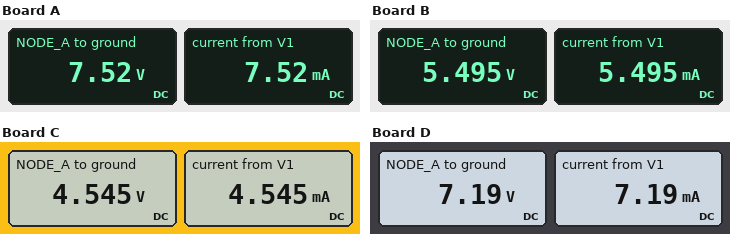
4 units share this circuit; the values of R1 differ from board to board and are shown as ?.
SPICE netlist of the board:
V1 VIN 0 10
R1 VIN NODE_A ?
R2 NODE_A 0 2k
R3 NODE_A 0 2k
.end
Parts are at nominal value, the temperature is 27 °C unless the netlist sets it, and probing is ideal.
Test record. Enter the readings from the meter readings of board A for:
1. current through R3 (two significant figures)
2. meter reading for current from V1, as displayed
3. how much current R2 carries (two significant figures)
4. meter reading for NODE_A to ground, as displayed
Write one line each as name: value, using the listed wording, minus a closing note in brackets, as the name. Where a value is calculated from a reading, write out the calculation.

current through R3: (7.52 V) / 2 kΩ = 3.8 mA
meter reading for current from V1, as displayed: 7.52 mA
how much current R2 carries: (7.52 V) / 2 kΩ = 3.8 mA
meter reading for NODE_A to ground, as displayed: 7.52 V
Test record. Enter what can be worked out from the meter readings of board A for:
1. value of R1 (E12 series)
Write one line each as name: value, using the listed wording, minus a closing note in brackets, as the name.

value of R1: 330 Ω
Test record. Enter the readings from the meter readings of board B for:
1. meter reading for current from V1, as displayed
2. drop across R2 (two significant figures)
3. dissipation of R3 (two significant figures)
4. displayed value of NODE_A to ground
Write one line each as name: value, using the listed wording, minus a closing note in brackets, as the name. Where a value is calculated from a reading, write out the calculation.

meter reading for current from V1, as displayed: 5.495 mA
drop across R2: 5.495 V = 5.5 V
dissipation of R3: (5.495 V)^2 / 2 kΩ = 15 mW
displayed value of NODE_A to ground: 5.495 V
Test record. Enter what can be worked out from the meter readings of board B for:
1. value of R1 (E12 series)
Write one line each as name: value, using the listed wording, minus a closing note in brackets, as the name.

value of R1: 820 Ω
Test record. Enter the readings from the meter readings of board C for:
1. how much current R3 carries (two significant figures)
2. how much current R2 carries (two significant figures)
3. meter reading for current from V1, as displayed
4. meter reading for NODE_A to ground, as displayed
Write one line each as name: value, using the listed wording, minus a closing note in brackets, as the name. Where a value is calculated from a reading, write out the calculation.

how much current R3 carries: (4.545 V) / 2 kΩ = 2.3 mA
how much current R2 carries: (4.545 V) / 2 kΩ = 2.3 mA
meter reading for current from V1, as displayed: 4.545 mA
meter reading for NODE_A to ground, as displayed: 4.545 V
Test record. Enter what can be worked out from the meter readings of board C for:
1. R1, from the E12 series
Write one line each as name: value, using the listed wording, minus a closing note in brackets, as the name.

R1, from the E12 series: 1.2 kΩ
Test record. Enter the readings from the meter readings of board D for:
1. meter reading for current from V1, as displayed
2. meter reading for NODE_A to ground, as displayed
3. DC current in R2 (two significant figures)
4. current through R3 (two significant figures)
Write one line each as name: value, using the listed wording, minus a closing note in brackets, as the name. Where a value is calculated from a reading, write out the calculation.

meter reading for current from V1, as displayed: 7.19 mA
meter reading for NODE_A to ground, as displayed: 7.19 V
DC current in R2: (7.19 V) / 2 kΩ = 3.6 mA
current through R3: (7.19 V) / 2 kΩ = 3.6 mA
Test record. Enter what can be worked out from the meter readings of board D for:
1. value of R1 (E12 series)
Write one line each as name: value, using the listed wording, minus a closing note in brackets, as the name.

value of R1: 390 Ω
